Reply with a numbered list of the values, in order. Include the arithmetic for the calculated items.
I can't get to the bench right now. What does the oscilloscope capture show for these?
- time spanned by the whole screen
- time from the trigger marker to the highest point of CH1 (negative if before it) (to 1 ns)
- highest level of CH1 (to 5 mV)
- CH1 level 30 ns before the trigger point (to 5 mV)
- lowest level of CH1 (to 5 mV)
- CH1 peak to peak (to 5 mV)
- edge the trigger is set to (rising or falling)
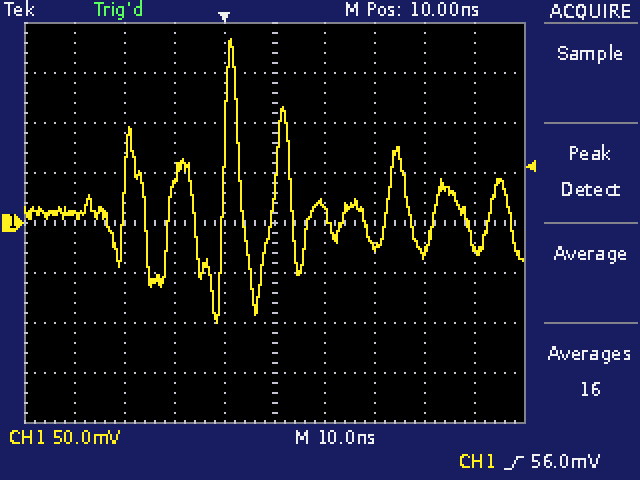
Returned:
1. 100 ns
2. +1 ns
3. 185 mV
4. 10 mV
5. -100 mV
6. 185 mV − (-100 mV) = 285 mV
7. rising
